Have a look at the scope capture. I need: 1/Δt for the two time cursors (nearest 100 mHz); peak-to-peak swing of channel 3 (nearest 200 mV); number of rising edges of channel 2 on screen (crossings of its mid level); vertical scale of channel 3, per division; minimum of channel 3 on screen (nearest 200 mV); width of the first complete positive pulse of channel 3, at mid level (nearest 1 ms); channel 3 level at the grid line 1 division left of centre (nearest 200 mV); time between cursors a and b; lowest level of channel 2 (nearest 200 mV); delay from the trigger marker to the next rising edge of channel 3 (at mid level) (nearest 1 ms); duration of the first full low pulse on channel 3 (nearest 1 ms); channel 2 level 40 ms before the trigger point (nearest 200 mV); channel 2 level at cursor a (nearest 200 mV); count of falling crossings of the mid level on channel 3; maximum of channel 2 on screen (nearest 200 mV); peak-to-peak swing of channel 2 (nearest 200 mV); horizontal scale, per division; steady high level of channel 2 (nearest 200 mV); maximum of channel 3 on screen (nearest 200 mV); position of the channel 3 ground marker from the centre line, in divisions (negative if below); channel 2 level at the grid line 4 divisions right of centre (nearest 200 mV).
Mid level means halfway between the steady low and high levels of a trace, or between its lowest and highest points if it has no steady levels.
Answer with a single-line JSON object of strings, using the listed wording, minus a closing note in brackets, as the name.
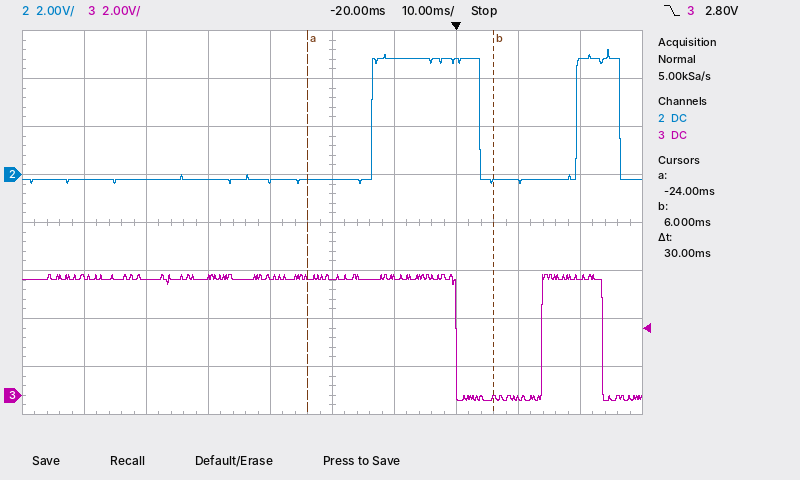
{"1/Δt for the two time cursors": "33.3 Hz", "peak-to-peak swing of channel 3": "5.2 V", "number of rising edges of channel 2 on screen": "2", "vertical scale of channel 3, per division": "2 V", "minimum of channel 3 on screen": "-200 mV", "width of the first complete positive pulse of channel 3, at mid level": "10 ms", "channel 3 level at the grid line 1 division left of centre": "5.0 V", "time between cursors a and b": "30 ms", "lowest level of channel 2": "-400 mV", "delay from the trigger marker to the next rising edge of channel 3 (at mid level)": "14 ms", "duration of the first full low pulse on channel 3": "14 ms", "channel 2 level 40 ms before the trigger point": "-200 mV", "channel 2 level at cursor a": "-200 mV", "count of falling crossings of the mid level on channel 3": "2", "maximum of channel 2 on screen": "5.2 V", "peak-to-peak swing of channel 2": "5.6 V", "horizontal scale, per division": "10 ms", "steady high level of channel 2": "4.8 V", "maximum of channel 3 on screen": "5.0 V", "position of the channel 3 ground marker from the centre line, in divisions": "-3.6 div", "channel 2 level at the grid line 4 divisions right of centre": "4.6 V"}
